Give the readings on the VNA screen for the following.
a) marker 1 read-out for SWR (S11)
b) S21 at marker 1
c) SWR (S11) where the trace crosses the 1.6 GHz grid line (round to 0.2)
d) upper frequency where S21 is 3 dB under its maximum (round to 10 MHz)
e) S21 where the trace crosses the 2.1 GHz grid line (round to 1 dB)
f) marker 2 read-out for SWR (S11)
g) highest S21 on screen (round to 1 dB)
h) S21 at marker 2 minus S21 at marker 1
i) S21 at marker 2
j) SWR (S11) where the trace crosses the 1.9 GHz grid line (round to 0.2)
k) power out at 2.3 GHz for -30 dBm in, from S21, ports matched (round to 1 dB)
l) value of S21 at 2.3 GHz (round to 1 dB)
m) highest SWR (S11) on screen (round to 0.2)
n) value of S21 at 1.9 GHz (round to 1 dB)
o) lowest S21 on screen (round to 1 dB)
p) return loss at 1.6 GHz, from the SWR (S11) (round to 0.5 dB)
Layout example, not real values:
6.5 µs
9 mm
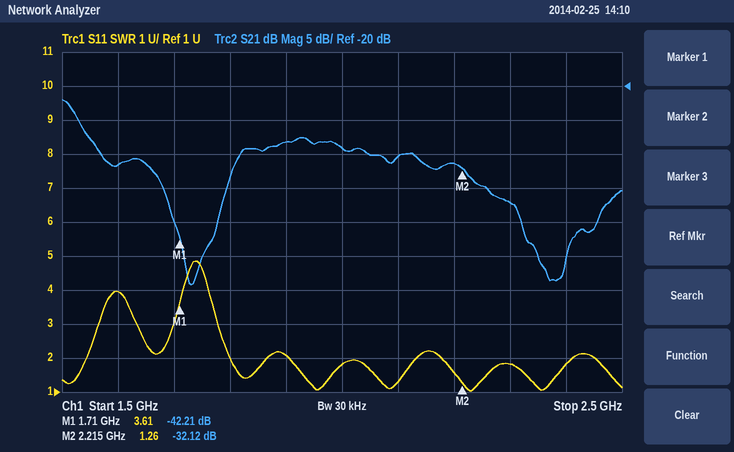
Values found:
3.61
-42.21 dB
4.0
1.53 GHz
-30 dB
1.26
-22 dB
10.09 dB
-32.12 dB
2.0
-67 dBm
-37 dB
4.8
-28 dB
-49 dB
4.5 dB
